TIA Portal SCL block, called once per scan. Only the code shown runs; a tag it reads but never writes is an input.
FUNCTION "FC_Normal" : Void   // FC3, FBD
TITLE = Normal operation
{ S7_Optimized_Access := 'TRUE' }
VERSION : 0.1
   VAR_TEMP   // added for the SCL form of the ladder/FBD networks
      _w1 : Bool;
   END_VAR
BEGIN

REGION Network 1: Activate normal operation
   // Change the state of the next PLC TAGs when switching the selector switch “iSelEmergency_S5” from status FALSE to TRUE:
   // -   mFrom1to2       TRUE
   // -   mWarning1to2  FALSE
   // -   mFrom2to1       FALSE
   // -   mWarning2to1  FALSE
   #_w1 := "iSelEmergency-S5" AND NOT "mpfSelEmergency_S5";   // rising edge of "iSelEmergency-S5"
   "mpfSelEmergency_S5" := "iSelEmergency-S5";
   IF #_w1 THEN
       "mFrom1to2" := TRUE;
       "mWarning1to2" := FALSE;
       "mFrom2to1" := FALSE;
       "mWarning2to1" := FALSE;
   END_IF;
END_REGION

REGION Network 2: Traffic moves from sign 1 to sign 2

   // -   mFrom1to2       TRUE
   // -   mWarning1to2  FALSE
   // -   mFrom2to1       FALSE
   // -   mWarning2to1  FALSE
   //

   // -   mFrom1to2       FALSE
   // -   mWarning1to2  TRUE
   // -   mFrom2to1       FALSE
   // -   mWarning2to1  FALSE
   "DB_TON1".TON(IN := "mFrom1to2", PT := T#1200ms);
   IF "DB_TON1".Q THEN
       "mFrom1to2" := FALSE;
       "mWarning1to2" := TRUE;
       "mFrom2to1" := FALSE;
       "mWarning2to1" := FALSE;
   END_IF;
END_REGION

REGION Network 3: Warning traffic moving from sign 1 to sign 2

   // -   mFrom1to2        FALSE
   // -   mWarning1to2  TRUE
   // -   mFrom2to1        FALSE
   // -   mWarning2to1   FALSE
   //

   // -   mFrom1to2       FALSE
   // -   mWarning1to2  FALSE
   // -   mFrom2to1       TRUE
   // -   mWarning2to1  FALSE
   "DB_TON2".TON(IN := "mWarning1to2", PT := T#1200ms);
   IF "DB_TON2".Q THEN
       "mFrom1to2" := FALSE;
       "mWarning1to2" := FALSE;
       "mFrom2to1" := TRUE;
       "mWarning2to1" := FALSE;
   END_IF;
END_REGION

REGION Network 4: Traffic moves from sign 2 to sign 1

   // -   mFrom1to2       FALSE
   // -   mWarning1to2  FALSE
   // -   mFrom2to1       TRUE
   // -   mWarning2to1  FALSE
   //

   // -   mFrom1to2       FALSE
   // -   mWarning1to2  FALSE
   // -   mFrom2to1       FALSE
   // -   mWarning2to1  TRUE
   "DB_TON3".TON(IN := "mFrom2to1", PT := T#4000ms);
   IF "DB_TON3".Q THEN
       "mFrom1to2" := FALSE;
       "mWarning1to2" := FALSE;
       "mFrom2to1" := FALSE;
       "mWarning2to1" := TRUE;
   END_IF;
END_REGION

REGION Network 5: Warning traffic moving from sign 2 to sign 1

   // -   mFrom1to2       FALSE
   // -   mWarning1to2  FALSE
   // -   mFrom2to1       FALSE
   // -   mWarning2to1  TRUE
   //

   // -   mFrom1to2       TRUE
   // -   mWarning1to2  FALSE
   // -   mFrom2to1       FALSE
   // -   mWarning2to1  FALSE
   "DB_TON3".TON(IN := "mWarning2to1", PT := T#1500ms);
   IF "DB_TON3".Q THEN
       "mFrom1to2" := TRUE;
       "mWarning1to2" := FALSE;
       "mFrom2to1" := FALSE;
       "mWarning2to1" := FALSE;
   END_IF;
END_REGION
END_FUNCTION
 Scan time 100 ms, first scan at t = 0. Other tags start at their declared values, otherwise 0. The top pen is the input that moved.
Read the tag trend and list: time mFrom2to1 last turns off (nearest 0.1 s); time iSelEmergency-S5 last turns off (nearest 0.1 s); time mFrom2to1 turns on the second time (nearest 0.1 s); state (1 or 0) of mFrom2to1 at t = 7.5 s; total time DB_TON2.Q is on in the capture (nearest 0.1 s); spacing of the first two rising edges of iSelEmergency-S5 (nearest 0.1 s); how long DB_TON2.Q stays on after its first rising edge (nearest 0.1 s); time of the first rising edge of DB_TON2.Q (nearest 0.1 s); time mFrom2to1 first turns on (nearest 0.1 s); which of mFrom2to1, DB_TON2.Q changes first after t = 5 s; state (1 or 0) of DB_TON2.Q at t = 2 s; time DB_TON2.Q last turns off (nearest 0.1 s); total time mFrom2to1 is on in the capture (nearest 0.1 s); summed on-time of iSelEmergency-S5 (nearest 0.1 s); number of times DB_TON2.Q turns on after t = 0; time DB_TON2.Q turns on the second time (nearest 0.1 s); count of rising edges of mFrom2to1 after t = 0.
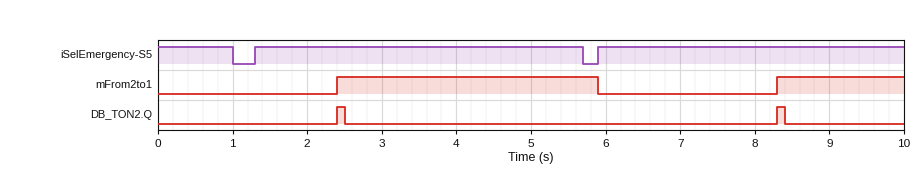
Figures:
5.9 s
5.7 s
8.3 s
0
0.2 s
4.6 s
0.1 s
2.4 s
2.4 s
mFrom2to1
0
8.4 s
5.2 s
9.5 s
2
8.3 s
2
